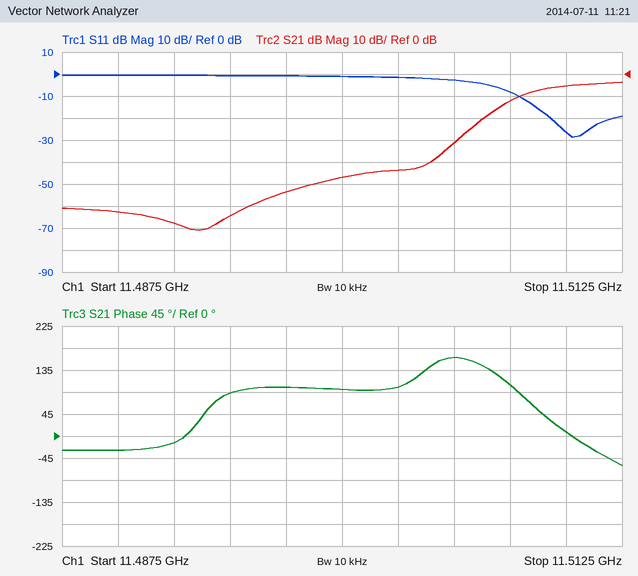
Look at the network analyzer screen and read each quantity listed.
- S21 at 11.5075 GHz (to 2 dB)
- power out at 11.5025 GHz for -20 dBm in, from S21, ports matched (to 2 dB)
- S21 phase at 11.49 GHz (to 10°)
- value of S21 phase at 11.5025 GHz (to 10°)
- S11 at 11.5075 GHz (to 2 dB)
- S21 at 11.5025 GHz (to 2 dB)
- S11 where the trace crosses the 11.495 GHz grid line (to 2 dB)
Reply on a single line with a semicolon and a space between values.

-12 dB; -64 dBm; -30°; 100°; -8 dB; -44 dB; 0 dB
